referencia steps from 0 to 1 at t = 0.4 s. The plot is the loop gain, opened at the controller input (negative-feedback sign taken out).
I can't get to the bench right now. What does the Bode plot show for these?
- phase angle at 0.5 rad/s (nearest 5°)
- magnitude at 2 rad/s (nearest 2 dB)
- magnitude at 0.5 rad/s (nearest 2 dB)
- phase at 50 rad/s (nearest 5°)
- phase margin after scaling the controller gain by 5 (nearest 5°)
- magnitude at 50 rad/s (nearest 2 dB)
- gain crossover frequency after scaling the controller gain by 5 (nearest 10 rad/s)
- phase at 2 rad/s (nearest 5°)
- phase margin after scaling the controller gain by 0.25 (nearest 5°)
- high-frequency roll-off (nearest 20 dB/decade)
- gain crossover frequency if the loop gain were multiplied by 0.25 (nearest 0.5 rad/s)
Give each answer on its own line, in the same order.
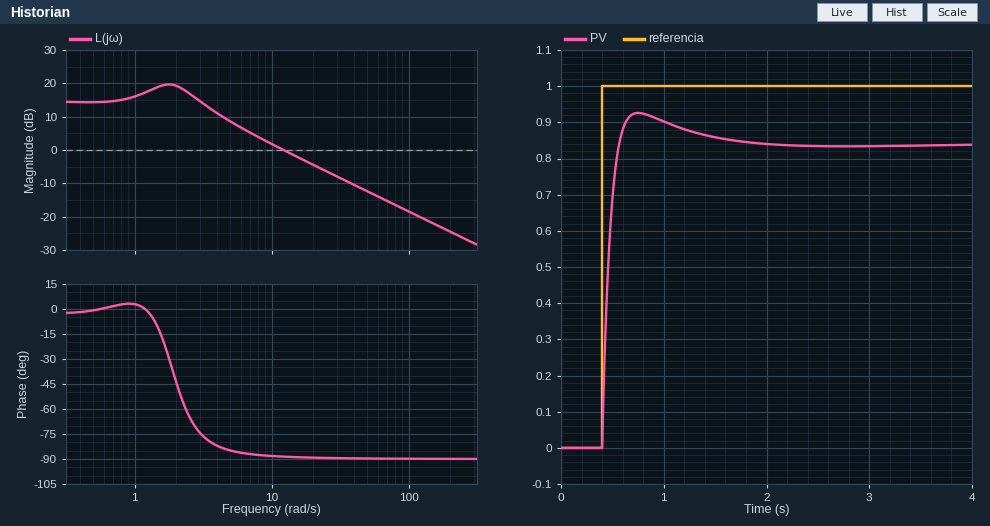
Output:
0°
20 dB
14 dB
-90°
90°
-12 dB
60 rad/s
-45°
100°
-20 dB/decade
3.5 rad/s
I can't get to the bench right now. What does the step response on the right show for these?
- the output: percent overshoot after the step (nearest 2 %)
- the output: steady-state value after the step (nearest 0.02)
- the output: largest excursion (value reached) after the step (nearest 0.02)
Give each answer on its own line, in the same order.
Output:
10 %
0.84
0.92
